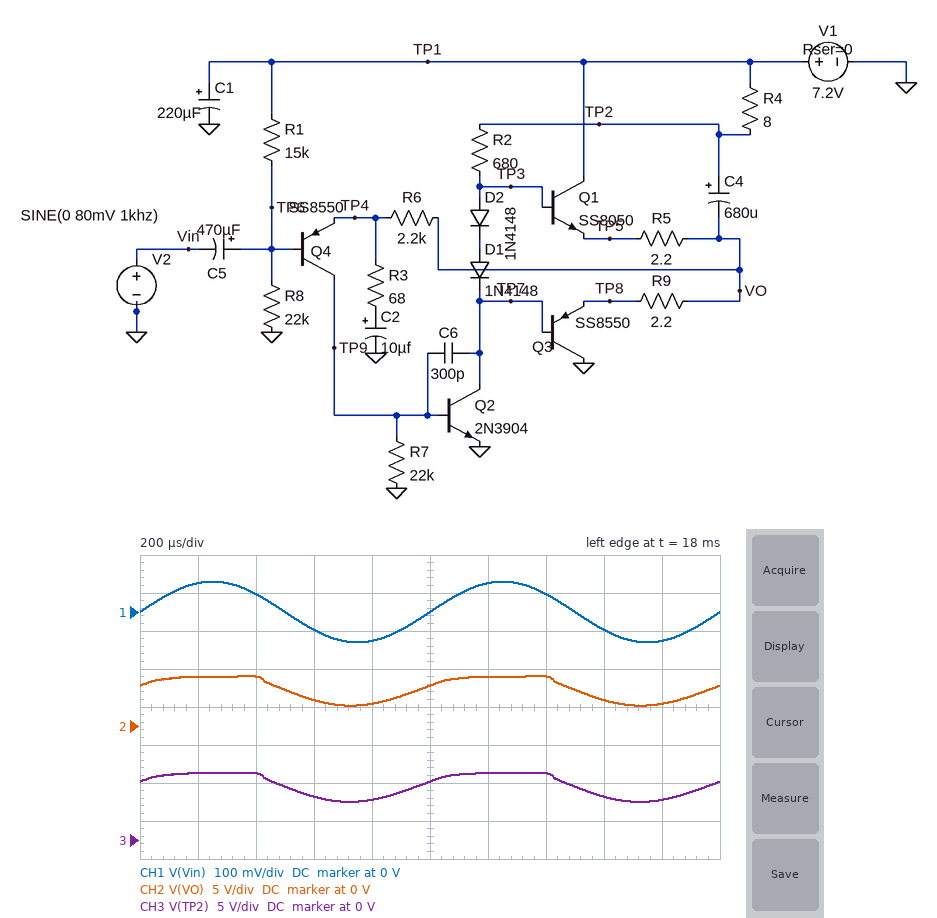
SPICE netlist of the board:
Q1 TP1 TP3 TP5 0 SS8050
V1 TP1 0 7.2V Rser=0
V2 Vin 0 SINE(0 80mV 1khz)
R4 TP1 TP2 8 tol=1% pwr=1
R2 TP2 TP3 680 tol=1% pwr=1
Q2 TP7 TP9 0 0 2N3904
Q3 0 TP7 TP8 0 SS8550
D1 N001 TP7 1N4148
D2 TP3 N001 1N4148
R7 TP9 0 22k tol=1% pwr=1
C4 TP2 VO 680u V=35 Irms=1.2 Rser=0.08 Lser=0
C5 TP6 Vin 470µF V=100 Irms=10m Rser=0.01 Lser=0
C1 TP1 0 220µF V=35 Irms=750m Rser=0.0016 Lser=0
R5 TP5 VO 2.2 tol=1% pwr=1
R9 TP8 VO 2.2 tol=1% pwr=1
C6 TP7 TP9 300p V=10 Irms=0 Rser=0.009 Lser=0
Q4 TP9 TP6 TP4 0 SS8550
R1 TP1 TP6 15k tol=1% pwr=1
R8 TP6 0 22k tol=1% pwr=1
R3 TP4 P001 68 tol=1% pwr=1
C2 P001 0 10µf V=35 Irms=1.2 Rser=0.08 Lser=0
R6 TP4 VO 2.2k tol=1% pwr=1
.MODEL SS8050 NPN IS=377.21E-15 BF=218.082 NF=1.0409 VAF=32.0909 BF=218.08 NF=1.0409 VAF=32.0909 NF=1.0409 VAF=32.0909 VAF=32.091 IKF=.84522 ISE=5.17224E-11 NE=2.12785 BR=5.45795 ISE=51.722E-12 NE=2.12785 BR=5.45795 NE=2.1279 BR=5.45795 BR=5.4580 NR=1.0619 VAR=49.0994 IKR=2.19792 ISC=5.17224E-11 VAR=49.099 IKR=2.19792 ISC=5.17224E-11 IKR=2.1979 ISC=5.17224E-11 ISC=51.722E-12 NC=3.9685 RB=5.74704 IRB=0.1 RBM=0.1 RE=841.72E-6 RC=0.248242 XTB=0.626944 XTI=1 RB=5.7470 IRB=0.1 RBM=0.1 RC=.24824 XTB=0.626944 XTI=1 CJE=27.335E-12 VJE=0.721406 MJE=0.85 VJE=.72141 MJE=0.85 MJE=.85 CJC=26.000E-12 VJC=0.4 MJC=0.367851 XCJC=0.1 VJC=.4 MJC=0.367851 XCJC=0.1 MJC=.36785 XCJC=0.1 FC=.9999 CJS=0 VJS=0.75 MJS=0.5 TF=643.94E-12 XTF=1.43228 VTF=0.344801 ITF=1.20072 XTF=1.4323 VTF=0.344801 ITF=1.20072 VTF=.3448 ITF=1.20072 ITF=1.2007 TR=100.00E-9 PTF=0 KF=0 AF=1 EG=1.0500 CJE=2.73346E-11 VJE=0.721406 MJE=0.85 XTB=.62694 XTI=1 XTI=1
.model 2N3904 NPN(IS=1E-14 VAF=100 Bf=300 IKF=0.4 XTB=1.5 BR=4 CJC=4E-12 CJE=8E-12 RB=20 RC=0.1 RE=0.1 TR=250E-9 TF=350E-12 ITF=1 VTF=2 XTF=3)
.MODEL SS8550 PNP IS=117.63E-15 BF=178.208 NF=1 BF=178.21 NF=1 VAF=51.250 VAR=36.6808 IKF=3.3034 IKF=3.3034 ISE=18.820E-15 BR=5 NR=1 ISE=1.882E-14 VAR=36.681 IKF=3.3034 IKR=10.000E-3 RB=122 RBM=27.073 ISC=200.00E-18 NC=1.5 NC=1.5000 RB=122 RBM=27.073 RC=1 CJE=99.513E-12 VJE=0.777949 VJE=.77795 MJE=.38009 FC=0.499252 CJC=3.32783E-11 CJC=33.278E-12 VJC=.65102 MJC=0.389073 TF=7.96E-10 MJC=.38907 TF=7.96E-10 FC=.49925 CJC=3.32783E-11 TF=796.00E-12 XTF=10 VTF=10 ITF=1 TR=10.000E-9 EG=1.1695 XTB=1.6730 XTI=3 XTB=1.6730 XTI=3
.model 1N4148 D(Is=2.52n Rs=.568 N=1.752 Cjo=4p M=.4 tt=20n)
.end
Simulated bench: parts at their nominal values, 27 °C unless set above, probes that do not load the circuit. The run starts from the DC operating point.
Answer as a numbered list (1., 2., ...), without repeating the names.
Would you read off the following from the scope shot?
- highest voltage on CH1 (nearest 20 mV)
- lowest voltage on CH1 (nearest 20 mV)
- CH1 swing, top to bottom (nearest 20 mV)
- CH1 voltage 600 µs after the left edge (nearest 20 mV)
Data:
1. 80 mV
2. -80 mV
3. 160 mV
4. -40 mV
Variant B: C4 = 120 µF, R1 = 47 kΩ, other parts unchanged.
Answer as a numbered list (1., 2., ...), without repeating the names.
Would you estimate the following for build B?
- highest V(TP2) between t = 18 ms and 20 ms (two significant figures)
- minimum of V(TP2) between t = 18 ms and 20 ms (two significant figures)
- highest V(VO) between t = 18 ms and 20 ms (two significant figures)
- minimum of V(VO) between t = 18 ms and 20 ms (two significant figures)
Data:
1. 9.3 V
2. 5.5 V
3. 5.2 V
4. 1.3 V
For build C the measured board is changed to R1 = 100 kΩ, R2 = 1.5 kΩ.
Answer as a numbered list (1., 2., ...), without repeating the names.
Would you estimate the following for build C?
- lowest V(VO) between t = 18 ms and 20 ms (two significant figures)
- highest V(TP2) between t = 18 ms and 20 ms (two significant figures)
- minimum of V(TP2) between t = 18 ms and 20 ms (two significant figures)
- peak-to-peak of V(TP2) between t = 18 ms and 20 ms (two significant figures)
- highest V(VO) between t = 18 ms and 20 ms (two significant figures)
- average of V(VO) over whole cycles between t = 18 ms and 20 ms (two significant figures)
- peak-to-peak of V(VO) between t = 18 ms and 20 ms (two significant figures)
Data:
1. 1.1 V
2. 9.0 V
3. 6.2 V
4. 2.7 V
5. 3.9 V
6. 2.1 V
7. 2.8 V
